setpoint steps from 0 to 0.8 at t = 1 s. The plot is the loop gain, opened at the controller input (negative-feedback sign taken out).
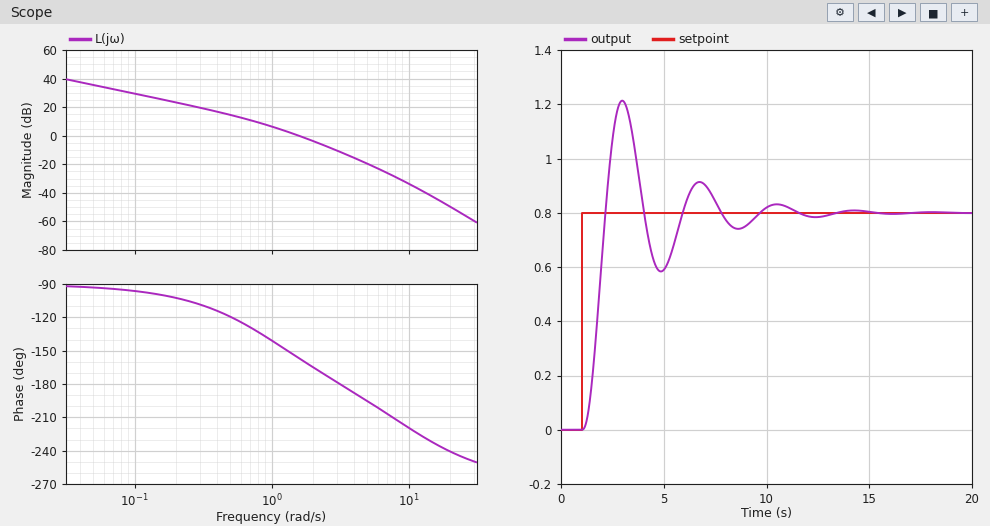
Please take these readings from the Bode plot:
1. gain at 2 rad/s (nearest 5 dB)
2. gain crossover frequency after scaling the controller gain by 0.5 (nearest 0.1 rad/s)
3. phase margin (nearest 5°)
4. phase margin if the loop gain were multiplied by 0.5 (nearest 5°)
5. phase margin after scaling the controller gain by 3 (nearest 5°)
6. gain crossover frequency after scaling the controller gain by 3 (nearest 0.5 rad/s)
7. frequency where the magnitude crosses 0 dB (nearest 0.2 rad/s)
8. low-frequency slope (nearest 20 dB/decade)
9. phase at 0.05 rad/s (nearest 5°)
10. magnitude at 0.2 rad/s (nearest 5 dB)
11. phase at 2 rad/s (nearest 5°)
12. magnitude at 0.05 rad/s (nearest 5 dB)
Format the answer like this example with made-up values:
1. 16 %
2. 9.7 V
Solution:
1. -5 dB
2. 1.0 rad/s
3. 25°
4. 40°
5. 5°
6. 3.0 rad/s
7. 1.6 rad/s
8. -20 dB/decade
9. -95°
10. 25 dB
11. -165°
12. 35 dB
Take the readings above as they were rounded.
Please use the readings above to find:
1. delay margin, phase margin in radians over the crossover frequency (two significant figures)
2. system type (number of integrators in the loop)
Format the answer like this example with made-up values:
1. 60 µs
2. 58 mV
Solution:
1. 0.27 s
2. 1
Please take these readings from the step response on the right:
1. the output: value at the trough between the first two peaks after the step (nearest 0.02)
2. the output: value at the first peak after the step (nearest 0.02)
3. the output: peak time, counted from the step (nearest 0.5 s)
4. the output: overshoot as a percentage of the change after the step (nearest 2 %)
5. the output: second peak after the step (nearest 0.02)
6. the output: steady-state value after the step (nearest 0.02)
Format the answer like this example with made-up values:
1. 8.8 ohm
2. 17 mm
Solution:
1. 0.58
2. 1.22
3. 2.0 s
4. 52 %
5. 0.92
6. 0.80
